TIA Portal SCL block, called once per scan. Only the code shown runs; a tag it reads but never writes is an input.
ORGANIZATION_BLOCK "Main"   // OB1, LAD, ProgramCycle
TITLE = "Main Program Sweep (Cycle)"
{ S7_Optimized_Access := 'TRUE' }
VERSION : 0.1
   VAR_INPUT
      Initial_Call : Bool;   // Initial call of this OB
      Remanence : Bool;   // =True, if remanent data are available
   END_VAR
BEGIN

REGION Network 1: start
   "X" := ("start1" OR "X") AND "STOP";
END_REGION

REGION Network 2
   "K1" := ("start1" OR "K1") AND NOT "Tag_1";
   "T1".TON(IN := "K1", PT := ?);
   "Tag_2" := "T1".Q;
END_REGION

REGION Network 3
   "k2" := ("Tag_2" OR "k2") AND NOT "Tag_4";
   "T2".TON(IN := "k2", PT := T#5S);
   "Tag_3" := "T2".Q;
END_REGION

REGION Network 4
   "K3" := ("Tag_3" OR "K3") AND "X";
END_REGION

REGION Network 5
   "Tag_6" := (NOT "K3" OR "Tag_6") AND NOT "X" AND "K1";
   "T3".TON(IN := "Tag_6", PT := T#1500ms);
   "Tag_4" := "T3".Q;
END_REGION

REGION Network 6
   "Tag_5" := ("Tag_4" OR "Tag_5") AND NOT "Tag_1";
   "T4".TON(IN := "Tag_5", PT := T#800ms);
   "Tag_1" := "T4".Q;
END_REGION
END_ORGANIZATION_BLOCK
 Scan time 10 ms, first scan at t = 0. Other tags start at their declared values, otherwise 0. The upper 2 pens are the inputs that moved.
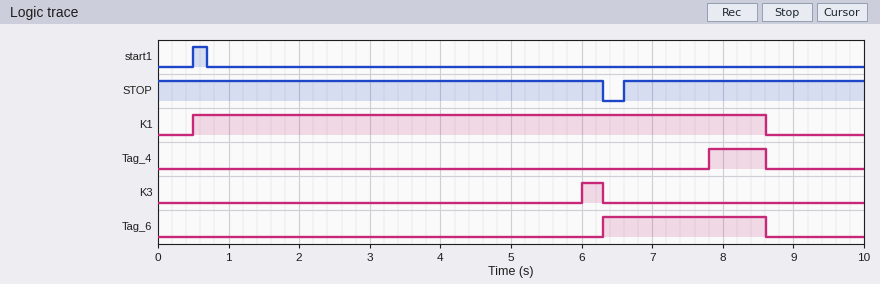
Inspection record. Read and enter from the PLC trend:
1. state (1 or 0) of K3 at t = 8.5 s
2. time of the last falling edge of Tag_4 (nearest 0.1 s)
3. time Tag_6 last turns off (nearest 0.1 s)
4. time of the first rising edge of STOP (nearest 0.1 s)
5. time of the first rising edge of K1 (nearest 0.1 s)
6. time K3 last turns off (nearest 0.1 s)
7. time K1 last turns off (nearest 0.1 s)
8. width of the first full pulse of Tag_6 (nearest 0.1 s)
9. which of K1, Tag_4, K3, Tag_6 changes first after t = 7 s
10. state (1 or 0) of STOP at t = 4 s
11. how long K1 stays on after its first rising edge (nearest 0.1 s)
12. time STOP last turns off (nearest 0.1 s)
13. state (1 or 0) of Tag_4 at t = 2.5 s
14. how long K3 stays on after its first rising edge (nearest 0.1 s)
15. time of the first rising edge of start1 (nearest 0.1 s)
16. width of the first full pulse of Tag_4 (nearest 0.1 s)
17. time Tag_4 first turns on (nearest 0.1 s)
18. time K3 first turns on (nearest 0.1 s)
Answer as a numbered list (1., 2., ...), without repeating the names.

1. 0
2. 8.6 s
3. 8.6 s
4. 6.6 s
5. 0.5 s
6. 6.3 s
7. 8.6 s
8. 2.3 s
9. Tag_4
10. 1
11. 8.1 s
12. 6.3 s
13. 0
14. 0.3 s
15. 0.5 s
16. 0.8 s
17. 7.8 s
18. 6.0 s
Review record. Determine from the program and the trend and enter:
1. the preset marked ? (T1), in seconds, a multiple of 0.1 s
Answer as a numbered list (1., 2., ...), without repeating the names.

1. 0.5 s
